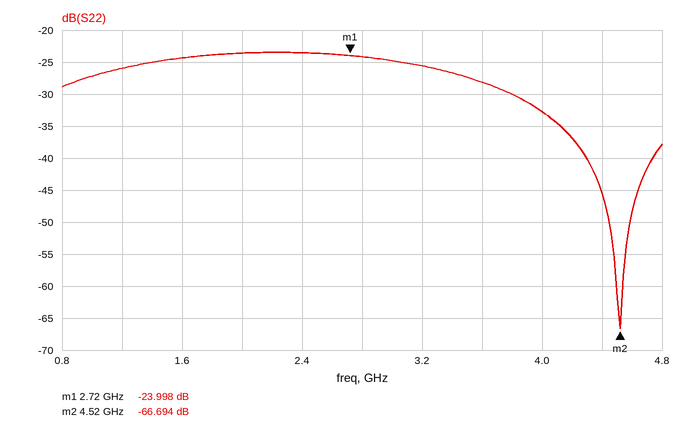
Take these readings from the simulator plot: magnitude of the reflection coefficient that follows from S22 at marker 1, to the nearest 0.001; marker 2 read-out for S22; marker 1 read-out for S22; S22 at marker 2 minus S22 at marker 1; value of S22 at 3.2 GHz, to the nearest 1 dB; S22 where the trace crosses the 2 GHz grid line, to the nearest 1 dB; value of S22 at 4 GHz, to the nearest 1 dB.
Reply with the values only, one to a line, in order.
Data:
0.063
-66.694 dB
-23.998 dB
-42.696 dB
-26 dB
-24 dB
-33 dB
